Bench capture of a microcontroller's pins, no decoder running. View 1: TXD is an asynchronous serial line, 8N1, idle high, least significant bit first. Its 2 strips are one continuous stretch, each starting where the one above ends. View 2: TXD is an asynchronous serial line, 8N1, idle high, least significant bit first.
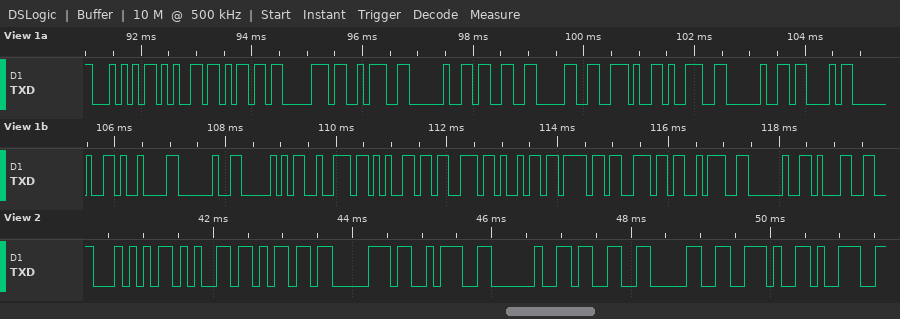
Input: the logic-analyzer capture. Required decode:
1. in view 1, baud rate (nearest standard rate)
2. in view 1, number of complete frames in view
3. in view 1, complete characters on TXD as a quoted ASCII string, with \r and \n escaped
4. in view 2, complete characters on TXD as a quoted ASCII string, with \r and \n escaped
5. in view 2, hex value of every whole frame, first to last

9600 baud
25
"Temp: 30.9 C \t Presion: 1"
"Temp: 30.9"
54 65 6D 70 3A 20 33 30 2E 39
